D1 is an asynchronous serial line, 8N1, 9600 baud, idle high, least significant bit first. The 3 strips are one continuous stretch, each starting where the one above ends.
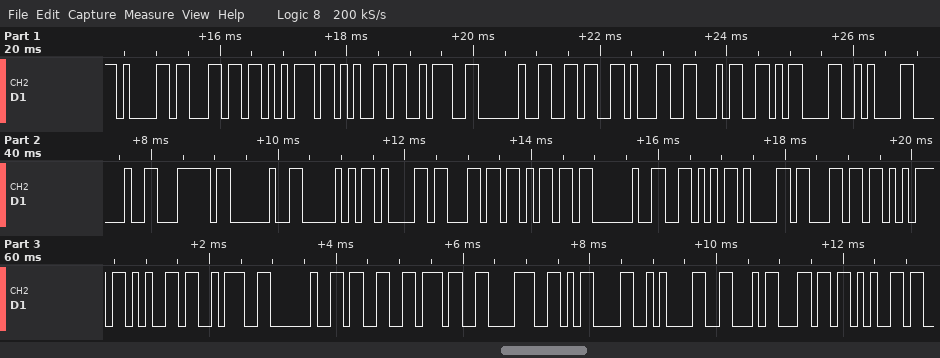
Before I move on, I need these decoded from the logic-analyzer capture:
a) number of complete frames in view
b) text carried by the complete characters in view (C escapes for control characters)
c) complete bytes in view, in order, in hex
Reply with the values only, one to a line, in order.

34
"alue: 614\r\n | Palm Value: 378\r\nFle"
0x61 0x6C 0x75 0x65 0x3A 0x20 0x36 0x31 0x34 0x0D 0x0A 0x20 0x7C 0x20 0x50 0x61 0x6C 0x6D 0x20 0x56 0x61 0x6C 0x75 0x65 0x3A 0x20 0x33 0x37 0x38 0x0D 0x0A 0x46 0x6C 0x65
